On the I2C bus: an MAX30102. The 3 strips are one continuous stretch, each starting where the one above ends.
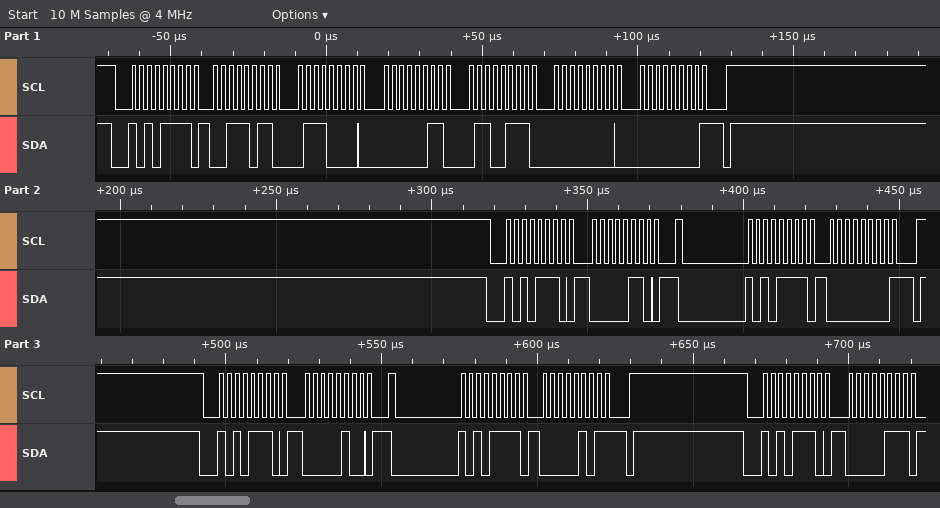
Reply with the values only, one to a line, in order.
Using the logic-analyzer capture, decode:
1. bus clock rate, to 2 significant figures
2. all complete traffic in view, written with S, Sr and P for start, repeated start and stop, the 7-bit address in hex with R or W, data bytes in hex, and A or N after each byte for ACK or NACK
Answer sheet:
400 kHz
S 57R A 3B A 70 A 03 A 67 A 00 A 00 N P S 57W A 06 A Sr 57R A 00 N P S 57W A 04 A Sr 57R A 05 N P S 57W A 07 A
